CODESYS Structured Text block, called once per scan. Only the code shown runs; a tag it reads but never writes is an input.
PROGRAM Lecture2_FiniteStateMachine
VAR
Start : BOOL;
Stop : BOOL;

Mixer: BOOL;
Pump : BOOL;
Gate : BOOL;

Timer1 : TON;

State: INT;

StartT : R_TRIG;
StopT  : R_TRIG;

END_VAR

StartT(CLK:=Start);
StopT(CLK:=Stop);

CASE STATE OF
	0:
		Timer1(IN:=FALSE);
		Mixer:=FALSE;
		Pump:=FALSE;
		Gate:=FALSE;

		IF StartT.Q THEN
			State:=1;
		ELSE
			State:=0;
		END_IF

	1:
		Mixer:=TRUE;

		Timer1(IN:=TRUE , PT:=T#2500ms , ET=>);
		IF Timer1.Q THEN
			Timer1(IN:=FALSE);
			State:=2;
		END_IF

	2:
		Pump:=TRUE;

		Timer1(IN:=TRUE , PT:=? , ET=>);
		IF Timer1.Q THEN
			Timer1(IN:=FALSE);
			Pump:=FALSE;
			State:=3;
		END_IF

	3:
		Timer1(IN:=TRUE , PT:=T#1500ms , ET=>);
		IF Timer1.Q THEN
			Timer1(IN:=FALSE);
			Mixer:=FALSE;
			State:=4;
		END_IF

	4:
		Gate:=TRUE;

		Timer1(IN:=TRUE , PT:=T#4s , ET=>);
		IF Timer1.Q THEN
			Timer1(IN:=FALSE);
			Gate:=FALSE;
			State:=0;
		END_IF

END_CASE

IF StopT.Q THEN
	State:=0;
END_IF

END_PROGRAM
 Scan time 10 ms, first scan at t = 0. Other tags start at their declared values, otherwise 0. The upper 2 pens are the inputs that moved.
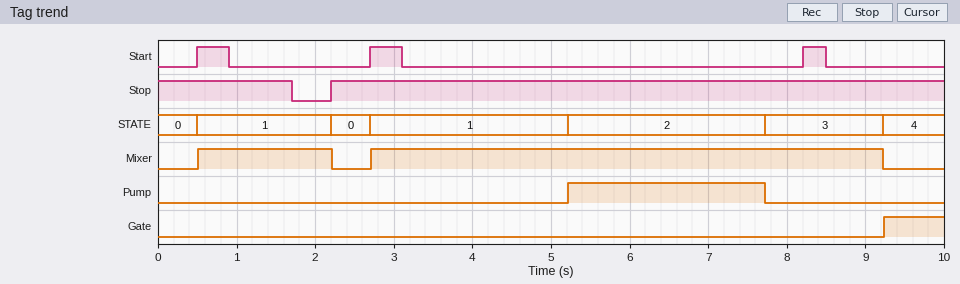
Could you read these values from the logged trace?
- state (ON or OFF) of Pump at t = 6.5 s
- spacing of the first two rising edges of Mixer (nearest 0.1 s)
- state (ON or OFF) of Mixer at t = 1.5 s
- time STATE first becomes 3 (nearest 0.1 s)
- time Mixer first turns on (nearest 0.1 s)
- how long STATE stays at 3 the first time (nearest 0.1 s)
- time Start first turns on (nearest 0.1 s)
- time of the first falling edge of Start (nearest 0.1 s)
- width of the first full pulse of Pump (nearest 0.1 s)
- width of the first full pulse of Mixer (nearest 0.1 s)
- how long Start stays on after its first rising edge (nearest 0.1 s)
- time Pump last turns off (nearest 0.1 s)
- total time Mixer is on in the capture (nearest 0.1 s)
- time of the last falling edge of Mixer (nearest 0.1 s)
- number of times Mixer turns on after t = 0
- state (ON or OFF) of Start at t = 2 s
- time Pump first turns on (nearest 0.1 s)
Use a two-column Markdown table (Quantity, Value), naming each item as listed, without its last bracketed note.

| Quantity | Value |
|---|---|
| state (ON or OFF) of Pump at t = 6.5 s | ON |
| spacing of the first two rising edges of Mixer | 2.2 s |
| state (ON or OFF) of Mixer at t = 1.5 s | ON |
| time STATE first becomes 3 | 7.7 s |
| time Mixer first turns on | 0.5 s |
| how long STATE stays at 3 the first time | 1.5 s |
| time Start first turns on | 0.5 s |
| time of the first falling edge of Start | 0.9 s |
| width of the first full pulse of Pump | 2.5 s |
| width of the first full pulse of Mixer | 1.7 s |
| how long Start stays on after its first rising edge | 0.4 s |
| time Pump last turns off | 7.7 s |
| total time Mixer is on in the capture | 8.2 s |
| time of the last falling edge of Mixer | 9.2 s |
| number of times Mixer turns on after t = 0 | 2 |
| state (ON or OFF) of Start at t = 2 s | OFF |
| time Pump first turns on | 5.2 s |
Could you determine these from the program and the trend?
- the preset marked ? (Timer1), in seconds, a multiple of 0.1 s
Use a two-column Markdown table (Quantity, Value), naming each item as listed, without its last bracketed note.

| Quantity | Value |
|---|---|
| the preset marked ? (Timer1), in seconds, a multiple of 0.1 s | 2.5 s |
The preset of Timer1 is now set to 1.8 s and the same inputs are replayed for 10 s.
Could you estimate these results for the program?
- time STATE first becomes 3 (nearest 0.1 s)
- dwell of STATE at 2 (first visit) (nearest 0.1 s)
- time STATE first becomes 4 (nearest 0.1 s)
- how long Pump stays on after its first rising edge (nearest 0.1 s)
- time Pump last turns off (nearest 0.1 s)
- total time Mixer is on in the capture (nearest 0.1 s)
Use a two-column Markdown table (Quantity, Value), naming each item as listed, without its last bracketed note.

| Quantity | Value |
|---|---|
| time STATE first becomes 3 | 7.0 s |
| dwell of STATE at 2 (first visit) | 1.8 s |
| time STATE first becomes 4 | 8.5 s |
| how long Pump stays on after its first rising edge | 1.8 s |
| time Pump last turns off | 7.0 s |
| total time Mixer is on in the capture | 7.5 s |
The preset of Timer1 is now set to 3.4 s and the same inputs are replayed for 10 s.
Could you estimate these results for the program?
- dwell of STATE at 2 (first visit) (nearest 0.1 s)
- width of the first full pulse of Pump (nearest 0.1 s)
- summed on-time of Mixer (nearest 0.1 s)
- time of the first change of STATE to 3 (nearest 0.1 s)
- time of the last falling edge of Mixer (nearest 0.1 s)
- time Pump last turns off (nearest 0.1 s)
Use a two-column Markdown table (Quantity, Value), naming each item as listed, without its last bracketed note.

| Quantity | Value |
|---|---|
| dwell of STATE at 2 (first visit) | 3.4 s |
| width of the first full pulse of Pump | 3.4 s |
| summed on-time of Mixer | 9.0 s |
| time of the first change of STATE to 3 | 8.6 s |
| time of the last falling edge of Mixer | 2.2 s |
| time Pump last turns off | 8.6 s |
